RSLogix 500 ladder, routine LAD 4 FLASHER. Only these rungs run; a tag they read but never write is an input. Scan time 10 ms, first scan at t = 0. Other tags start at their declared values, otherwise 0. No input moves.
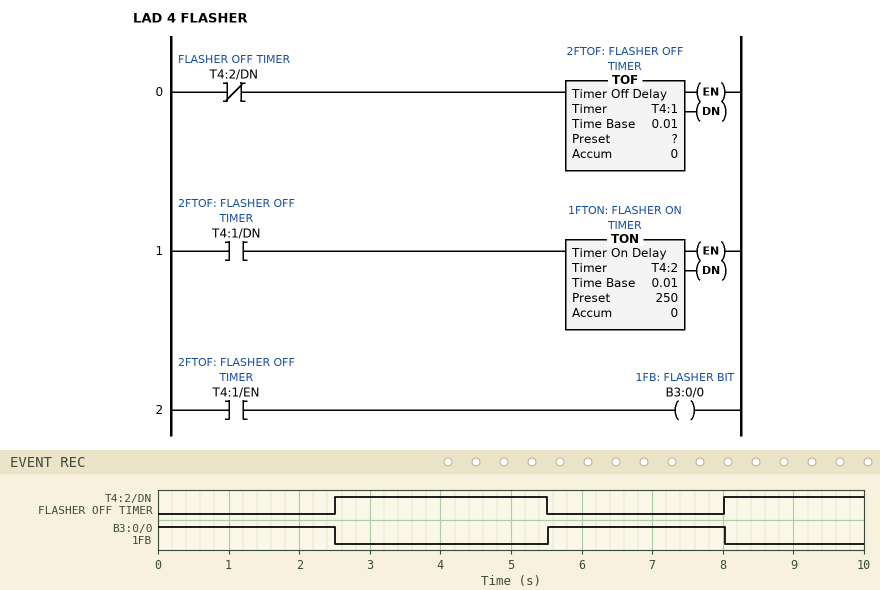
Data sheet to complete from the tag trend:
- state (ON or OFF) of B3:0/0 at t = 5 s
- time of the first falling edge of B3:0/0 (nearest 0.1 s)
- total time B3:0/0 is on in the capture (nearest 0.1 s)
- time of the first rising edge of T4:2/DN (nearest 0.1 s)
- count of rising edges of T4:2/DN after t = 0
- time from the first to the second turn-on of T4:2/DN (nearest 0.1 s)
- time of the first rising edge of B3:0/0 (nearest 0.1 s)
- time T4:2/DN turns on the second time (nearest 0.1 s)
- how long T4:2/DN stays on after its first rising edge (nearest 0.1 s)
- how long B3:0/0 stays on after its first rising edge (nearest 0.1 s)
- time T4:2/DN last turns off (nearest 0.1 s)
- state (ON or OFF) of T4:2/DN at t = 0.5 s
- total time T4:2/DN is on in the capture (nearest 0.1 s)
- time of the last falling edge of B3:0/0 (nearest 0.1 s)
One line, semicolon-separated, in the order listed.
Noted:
OFF; 2.5 s; 5.0 s; 2.5 s; 2; 5.5 s; 5.5 s; 8.0 s; 3.0 s; 2.5 s; 5.5 s; OFF; 5.0 s; 8.0 s
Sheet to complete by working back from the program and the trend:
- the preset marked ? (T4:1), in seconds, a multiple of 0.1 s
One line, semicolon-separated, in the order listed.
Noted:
3.0 s
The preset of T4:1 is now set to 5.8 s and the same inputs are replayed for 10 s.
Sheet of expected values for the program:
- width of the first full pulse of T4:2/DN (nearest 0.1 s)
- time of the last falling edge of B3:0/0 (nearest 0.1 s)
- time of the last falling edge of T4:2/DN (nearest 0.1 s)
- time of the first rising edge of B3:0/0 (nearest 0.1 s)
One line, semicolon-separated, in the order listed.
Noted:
5.8 s; 2.5 s; 8.3 s; 8.3 s
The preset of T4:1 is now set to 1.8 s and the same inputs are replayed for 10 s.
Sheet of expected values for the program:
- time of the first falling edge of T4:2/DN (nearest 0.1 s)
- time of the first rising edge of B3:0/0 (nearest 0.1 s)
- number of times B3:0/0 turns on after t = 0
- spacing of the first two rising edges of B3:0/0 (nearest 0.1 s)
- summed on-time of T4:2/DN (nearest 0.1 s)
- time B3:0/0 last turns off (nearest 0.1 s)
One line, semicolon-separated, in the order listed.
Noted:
4.3 s; 4.3 s; 2; 4.3 s; 3.6 s; 6.8 s
